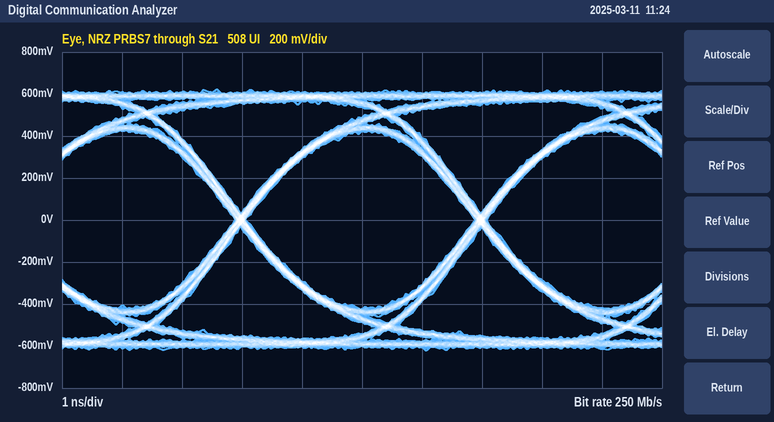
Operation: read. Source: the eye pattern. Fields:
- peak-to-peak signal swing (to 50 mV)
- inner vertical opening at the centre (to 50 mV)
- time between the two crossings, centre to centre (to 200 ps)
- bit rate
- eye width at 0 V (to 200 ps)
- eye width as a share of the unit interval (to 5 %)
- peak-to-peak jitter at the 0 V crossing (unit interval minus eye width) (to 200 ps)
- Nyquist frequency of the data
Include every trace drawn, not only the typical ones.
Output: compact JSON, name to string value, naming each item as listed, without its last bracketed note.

{"peak-to-peak signal swing": "1.25 V", "inner vertical opening at the centre": "850 mV", "time between the two crossings, centre to centre": "4.0 ns", "bit rate": "250 Mb/s", "eye width at 0 V": "3.8 ns", "eye width as a share of the unit interval": "95 %", "peak-to-peak jitter at the 0 V crossing (unit interval minus eye width)": "200 ps", "Nyquist frequency of the data": "125 MHz"}
